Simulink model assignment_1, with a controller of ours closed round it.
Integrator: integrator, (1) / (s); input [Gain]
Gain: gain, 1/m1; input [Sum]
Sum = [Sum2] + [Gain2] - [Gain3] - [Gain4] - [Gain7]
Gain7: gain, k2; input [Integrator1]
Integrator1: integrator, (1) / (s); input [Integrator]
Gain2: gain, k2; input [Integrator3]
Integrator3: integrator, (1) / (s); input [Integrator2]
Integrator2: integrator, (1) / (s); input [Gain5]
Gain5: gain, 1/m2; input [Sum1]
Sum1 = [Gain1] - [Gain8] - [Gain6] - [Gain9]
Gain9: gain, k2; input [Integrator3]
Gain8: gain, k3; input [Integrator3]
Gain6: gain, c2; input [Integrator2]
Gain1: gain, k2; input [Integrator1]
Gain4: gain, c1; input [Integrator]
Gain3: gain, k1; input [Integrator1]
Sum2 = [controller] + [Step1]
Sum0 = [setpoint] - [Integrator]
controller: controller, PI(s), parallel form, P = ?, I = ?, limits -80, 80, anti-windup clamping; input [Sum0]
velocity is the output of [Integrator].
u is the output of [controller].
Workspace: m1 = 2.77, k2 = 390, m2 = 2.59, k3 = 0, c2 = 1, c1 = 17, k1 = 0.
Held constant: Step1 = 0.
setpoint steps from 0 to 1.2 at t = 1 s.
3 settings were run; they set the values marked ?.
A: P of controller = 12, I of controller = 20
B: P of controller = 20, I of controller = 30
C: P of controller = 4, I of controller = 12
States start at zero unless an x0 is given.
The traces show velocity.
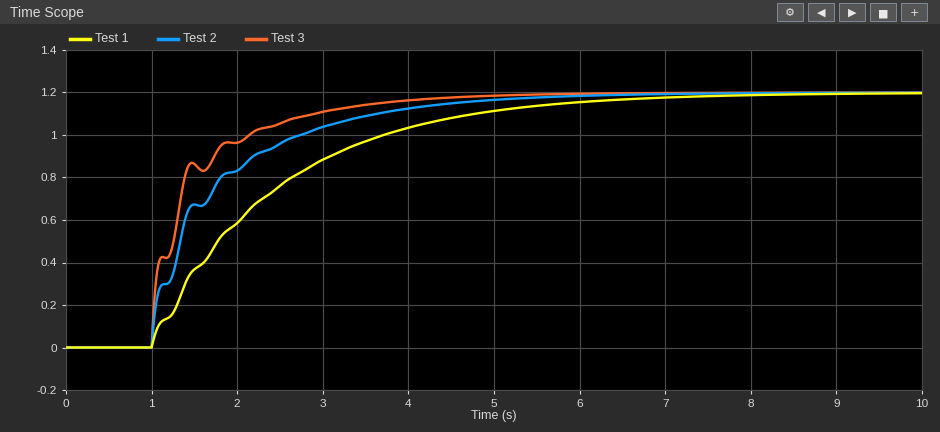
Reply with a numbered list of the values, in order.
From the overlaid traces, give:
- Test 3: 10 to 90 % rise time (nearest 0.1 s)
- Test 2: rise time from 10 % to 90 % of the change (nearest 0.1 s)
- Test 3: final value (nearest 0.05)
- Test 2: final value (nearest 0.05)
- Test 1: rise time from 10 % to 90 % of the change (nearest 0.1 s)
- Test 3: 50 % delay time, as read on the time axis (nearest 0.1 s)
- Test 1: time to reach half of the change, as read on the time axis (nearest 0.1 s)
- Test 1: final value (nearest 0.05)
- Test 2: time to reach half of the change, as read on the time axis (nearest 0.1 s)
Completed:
1. 1.7 s
2. 2.4 s
3. 1.20
4. 1.20
5. 3.4 s
6. 1.3 s
7. 2.0 s
8. 1.20
9. 1.4 s
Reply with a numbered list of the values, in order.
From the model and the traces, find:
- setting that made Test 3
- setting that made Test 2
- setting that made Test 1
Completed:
1. B
2. A
3. C
